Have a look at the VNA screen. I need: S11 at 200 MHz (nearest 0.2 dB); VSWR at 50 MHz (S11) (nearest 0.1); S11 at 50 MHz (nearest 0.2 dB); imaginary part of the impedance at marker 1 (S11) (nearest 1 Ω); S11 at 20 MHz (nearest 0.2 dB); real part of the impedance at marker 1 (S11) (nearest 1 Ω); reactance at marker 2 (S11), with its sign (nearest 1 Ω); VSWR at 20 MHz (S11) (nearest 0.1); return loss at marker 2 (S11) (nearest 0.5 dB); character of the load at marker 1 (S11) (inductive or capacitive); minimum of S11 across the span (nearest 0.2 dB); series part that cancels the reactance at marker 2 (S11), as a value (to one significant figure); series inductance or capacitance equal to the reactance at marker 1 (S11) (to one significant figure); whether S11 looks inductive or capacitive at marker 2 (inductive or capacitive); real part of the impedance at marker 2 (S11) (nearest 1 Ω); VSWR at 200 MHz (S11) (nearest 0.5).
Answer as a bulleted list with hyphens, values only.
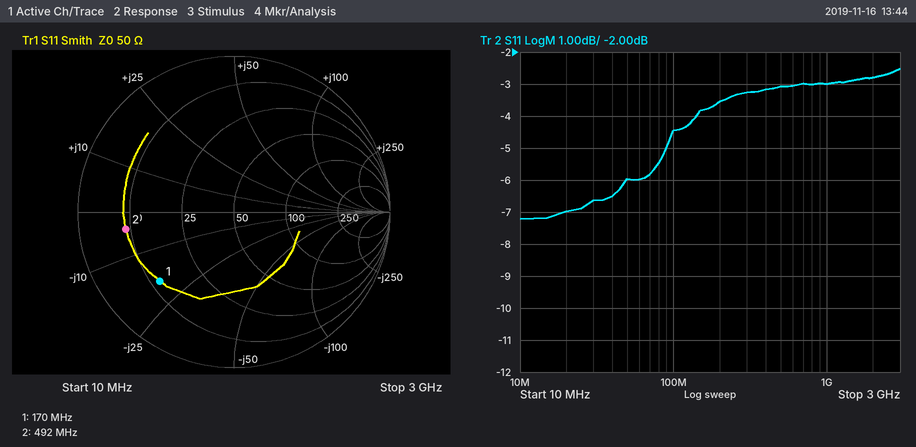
- -3.6 dB
- 3.0
- -6.0 dB
- -19 Ω
- -7.0 dB
- 12 Ω
- -4 Ω
- 2.6
- 3.0 dB
- capacitive
- -7.2 dB
- 1 nH
- 50 pF
- capacitive
- 9 Ω
- 5.0
